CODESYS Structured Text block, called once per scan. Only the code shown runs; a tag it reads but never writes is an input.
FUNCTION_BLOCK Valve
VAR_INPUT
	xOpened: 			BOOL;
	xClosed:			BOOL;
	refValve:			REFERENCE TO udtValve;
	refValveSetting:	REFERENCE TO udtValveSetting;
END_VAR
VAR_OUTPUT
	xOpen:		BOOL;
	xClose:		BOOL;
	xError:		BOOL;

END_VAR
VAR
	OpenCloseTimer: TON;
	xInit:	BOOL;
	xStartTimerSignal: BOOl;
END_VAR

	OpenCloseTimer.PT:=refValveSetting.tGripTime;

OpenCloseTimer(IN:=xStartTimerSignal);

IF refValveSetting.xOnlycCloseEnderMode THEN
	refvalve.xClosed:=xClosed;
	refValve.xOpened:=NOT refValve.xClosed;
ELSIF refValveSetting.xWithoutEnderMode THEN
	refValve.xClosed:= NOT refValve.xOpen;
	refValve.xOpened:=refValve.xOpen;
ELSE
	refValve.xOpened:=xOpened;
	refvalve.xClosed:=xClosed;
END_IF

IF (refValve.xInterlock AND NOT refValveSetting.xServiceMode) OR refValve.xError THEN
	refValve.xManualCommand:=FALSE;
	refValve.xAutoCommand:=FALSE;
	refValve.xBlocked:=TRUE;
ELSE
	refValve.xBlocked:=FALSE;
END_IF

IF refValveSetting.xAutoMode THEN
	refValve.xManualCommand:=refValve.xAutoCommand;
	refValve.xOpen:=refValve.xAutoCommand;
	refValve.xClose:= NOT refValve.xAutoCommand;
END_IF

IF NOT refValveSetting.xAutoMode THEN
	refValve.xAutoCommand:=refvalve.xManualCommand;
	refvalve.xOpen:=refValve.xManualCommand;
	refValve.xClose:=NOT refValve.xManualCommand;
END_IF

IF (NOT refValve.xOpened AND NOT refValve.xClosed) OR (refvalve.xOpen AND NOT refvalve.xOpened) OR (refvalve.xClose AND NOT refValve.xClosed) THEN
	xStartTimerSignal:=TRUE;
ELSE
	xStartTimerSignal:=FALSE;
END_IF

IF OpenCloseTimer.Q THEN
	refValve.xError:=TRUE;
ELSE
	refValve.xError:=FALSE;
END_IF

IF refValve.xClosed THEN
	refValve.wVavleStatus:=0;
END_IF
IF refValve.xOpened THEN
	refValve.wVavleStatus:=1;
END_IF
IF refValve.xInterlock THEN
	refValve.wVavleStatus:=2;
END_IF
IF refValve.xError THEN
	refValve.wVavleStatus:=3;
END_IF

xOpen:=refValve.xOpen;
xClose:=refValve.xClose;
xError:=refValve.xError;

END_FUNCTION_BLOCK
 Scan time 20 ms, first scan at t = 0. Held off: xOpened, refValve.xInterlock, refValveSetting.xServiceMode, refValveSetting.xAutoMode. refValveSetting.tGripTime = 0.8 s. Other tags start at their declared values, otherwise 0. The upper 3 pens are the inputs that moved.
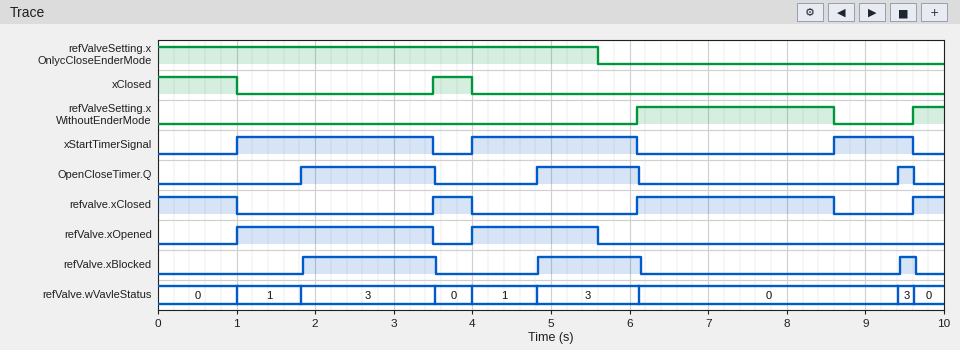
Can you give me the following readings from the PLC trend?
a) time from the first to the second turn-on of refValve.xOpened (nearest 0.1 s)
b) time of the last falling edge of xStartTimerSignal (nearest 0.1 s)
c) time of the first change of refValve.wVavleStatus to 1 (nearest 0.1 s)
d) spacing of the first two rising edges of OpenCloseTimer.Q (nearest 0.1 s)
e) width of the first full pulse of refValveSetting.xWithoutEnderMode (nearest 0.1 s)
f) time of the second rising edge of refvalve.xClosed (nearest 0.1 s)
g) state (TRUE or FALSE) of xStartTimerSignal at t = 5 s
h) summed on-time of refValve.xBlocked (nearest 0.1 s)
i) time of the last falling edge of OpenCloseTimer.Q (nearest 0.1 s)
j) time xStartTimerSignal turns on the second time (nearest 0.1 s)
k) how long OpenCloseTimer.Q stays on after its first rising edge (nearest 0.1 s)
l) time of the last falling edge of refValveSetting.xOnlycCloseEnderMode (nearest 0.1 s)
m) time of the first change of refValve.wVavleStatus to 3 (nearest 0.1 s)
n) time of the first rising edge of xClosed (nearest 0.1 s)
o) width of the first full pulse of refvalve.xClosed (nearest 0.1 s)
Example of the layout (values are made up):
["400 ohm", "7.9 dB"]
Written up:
["3.0 s", "9.6 s", "1.0 s", "3.0 s", "2.5 s", "6.1 s", "TRUE", "3.2 s", "9.6 s", "4.0 s", "1.7 s", "5.6 s", "1.8 s", "3.5 s", "0.5 s"]
